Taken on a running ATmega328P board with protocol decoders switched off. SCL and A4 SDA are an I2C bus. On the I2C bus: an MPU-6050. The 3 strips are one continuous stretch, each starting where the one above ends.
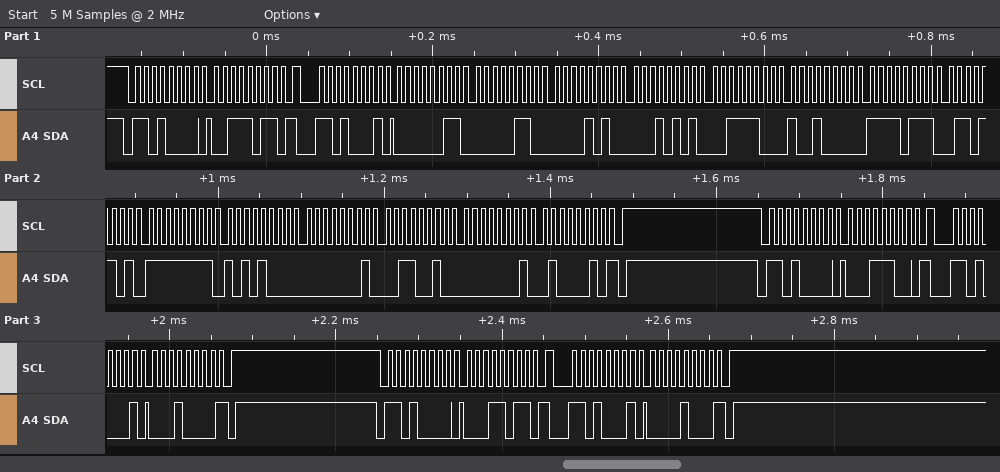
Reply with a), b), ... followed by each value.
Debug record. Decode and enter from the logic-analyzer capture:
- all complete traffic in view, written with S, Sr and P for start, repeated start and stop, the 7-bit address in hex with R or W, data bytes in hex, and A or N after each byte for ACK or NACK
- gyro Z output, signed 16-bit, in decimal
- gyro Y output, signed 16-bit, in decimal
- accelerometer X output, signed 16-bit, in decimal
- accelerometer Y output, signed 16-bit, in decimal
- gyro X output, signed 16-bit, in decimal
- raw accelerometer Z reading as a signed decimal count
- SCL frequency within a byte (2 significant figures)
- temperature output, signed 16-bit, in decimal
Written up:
a) S 68W A 3B A Sr 68R A 03 A 06 A 0A A 15 A 3C A 90 A F7 A 6D A FF A A8 A 01 A 32 A 01 A 42 N P S 68W A 1C A Sr 68R A 10 N P S 68W A 1B A Sr 68R A 08 N P
b) 322
c) 306
d) 774
e) 2581
f) -88
g) 15504
h) 100 kHz
i) -2195
